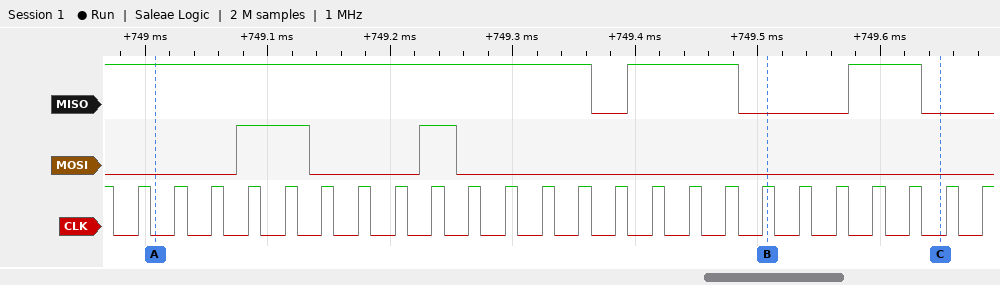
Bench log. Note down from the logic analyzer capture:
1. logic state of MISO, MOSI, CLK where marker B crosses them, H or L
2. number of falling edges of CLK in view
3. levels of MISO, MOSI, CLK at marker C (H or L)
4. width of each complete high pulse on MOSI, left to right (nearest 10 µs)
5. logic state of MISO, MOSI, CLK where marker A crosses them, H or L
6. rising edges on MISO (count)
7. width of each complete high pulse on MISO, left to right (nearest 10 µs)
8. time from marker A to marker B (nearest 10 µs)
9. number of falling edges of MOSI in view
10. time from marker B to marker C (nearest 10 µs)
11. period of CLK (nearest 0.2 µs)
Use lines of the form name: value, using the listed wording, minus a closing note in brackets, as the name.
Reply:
logic state of MISO, MOSI, CLK where marker B crosses them, H or L: MISO=L, MOSI=L, CLK=H
number of falling edges of CLK in view: 24
levels of MISO, MOSI, CLK at marker C: MISO=L, MOSI=L, CLK=L
width of each complete high pulse on MOSI, left to right: 60 µs, 30 µs
logic state of MISO, MOSI, CLK where marker A crosses them, H or L: MISO=H, MOSI=L, CLK=L
rising edges on MISO: 2
width of each complete high pulse on MISO, left to right: 90 µs, 60 µs
time from marker A to marker B: 500 µs
number of falling edges of MOSI in view: 2
time from marker B to marker C: 140 µs
period of CLK: 30 µs
